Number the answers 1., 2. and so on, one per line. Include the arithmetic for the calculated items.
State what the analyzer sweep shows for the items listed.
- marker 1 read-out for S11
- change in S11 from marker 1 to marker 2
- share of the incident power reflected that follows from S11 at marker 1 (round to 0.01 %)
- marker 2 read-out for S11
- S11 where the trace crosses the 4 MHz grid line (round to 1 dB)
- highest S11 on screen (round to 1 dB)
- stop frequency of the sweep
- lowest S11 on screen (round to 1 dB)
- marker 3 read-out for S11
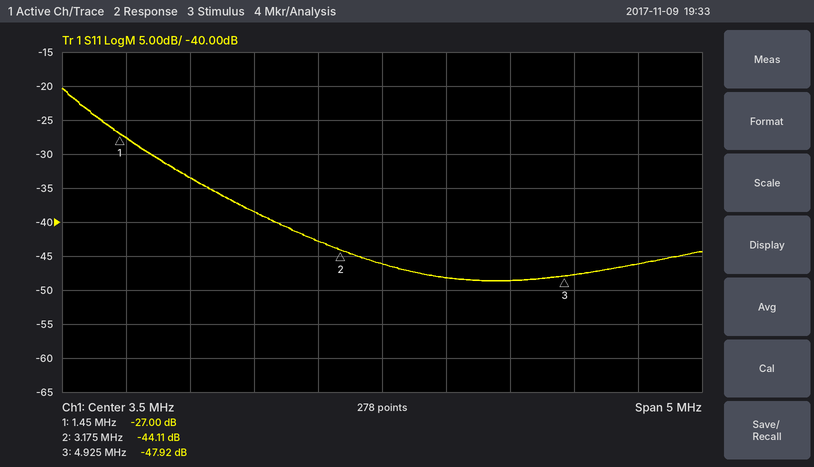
1. -27.00 dB
2. -44.11 − (-27) = -17.11 dB
3. 10^(-27/10) ≈ 0.20 %
4. -44.11 dB
5. -48 dB
6. -20 dB
7. 6 MHz
8. -49 dB
9. -47.92 dB
